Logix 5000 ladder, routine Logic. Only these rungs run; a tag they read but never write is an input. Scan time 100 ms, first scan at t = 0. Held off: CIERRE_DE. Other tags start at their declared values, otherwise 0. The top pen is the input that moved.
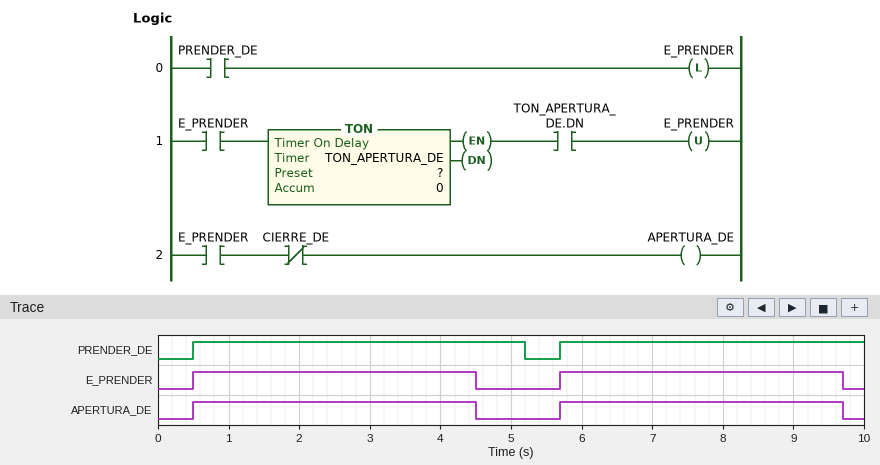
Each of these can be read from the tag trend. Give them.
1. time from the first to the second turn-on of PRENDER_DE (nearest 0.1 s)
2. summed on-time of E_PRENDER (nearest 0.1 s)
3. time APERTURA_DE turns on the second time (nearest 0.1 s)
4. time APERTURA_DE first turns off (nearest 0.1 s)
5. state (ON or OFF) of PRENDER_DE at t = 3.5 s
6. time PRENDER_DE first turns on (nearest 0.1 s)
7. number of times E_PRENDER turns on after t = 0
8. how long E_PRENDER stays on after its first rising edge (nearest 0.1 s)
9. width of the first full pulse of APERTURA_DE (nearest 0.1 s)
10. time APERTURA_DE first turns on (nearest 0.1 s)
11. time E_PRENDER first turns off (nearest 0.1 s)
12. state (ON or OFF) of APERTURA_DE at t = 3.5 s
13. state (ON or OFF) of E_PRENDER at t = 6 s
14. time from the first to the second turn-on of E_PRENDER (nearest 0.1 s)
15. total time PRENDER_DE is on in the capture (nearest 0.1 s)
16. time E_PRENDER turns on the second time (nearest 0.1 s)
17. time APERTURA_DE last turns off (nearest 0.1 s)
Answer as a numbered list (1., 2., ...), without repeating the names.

1. 5.2 s
2. 8.0 s
3. 5.7 s
4. 4.5 s
5. ON
6. 0.5 s
7. 2
8. 4.0 s
9. 4.0 s
10. 0.5 s
11. 4.5 s
12. ON
13. ON
14. 5.2 s
15. 9.0 s
16. 5.7 s
17. 9.7 s
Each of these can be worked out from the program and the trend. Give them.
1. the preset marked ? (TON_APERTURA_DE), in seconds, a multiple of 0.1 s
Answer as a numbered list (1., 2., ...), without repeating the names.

1. 4.0 s
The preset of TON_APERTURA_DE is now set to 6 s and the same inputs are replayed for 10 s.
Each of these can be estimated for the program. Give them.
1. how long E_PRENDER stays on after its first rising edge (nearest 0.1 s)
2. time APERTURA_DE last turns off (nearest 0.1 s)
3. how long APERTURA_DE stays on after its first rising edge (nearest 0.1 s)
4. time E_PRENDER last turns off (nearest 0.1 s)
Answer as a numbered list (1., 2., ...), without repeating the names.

1. 6.0 s
2. 6.5 s
3. 6.0 s
4. 6.5 s
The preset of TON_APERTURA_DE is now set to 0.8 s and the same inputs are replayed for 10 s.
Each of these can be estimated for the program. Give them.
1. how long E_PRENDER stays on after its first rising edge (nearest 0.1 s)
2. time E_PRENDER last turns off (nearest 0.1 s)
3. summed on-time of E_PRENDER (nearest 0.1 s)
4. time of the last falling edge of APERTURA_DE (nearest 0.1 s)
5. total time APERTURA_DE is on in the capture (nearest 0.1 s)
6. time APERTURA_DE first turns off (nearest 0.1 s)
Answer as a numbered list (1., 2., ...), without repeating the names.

1. 0.8 s
2. 6.5 s
3. 1.6 s
4. 6.5 s
5. 1.6 s
6. 1.3 s
